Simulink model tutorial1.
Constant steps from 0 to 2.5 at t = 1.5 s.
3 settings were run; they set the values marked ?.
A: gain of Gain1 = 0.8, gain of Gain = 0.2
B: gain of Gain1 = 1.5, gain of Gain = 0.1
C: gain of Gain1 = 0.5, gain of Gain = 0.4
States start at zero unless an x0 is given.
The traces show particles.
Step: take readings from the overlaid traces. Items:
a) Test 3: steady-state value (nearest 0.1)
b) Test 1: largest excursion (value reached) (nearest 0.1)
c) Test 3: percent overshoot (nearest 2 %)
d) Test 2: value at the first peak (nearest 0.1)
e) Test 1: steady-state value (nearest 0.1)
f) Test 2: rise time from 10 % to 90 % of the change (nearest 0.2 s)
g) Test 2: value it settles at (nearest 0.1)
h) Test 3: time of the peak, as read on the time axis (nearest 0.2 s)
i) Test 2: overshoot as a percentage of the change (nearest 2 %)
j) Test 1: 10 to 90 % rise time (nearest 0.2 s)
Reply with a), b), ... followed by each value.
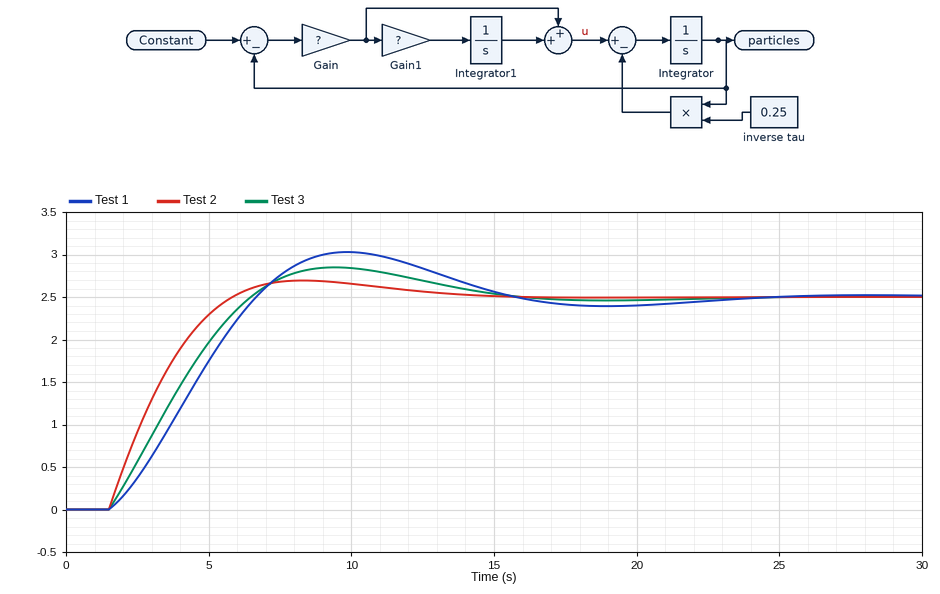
a) 2.5
b) 3.0
c) 14 %
d) 2.7
e) 2.5
f) 3.2 s
g) 2.5
h) 9.4 s
i) 8 %
j) 3.8 s
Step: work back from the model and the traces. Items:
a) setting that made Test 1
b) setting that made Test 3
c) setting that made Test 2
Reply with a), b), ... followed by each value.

a) B
b) A
c) C
